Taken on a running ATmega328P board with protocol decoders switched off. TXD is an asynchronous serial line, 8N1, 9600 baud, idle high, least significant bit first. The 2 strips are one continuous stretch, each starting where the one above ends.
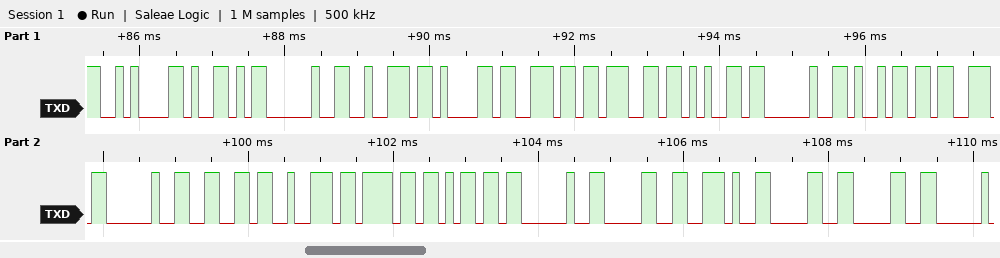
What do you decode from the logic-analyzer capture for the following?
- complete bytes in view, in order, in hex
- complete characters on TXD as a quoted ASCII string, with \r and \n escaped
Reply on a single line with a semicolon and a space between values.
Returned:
0x0A 0x59 0x20 0x72 0x61 0x6E 0x67 0x65 0x20 0x69 0x73 0x20 0x66 0x72 0x6F 0x6D 0x20 0x30 0x2E 0x30 0x30; "\nY range is from 0.00"
